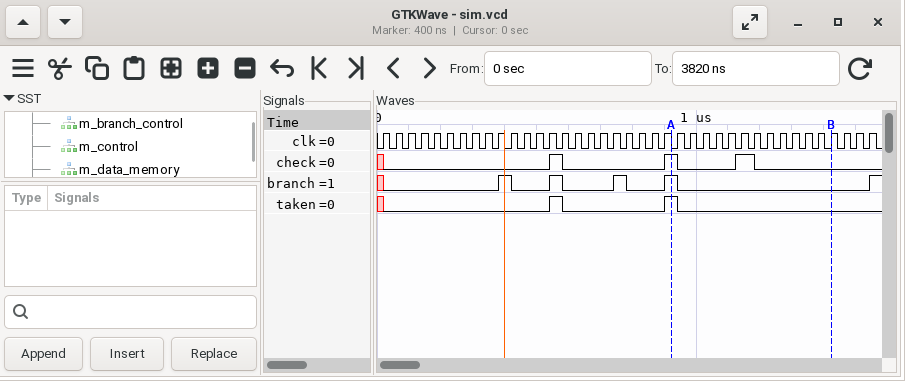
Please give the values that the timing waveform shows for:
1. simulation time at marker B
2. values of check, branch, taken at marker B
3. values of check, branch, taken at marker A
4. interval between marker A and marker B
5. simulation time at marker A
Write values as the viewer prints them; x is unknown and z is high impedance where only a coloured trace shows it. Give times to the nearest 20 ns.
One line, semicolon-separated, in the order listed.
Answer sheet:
1420 ns; check=0, branch=0, taken=0; check=1, branch=1, taken=1; 500 ns; 920 ns
